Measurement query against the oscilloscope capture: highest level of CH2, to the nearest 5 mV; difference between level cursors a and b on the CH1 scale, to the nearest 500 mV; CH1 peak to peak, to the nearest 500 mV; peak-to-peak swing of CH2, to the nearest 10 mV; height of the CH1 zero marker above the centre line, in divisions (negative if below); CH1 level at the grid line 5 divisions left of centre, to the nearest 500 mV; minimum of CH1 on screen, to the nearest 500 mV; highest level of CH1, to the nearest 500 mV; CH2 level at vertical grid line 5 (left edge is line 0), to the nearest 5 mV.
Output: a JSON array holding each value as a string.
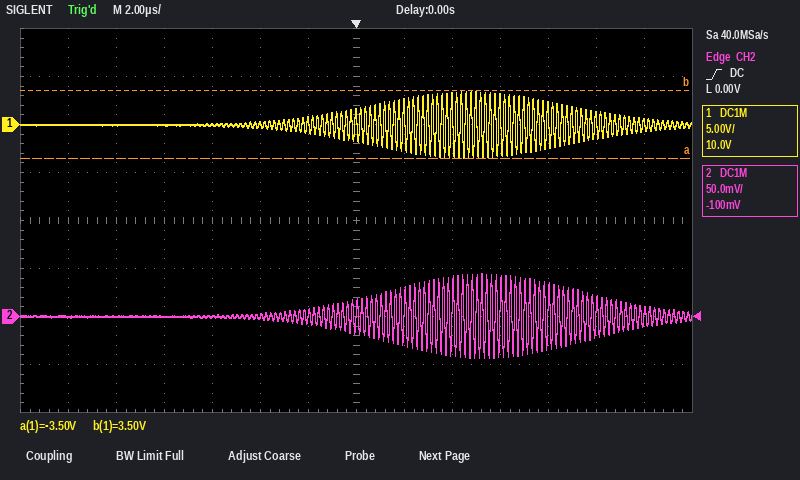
["45 mV", "7.0 V", "7.0 V", "90 mV", "+2.0 div", "0.0 V", "-3.5 V", "3.5 V", "0 mV"]
